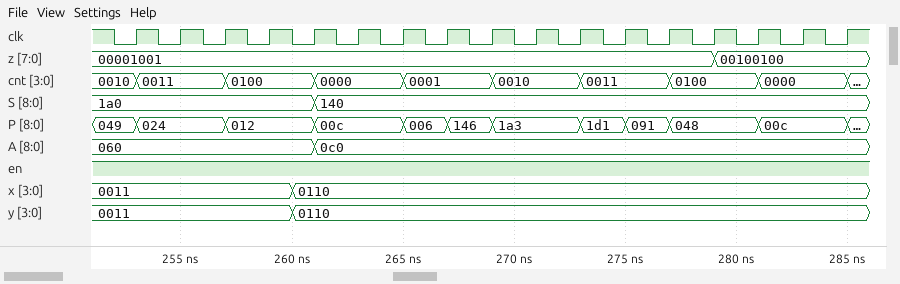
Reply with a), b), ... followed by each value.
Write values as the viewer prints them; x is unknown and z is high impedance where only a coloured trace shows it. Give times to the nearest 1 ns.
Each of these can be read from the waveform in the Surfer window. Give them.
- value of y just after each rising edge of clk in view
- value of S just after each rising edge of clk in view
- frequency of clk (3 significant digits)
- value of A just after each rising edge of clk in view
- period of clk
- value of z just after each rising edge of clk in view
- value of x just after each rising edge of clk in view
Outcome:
a) 0011, 0011, 0011, 0011, 0110, 0110, 0110, 0110, 0110, 0110, 0110, 0110, 0110, 0110, 0110, 0110, 0110
b) 1a0, 1a0, 1a0, 1a0, 140, 140, 140, 140, 140, 140, 140, 140, 140, 140, 140, 140, 140
c) 500 MHz
d) 060, 060, 060, 060, 0c0, 0c0, 0c0, 0c0, 0c0, 0c0, 0c0, 0c0, 0c0, 0c0, 0c0, 0c0, 0c0
e) 2 ns
f) 00001001, 00001001, 00001001, 00001001, 00001001, 00001001, 00001001, 00001001, 00001001, 00001001, 00001001, 00001001, 00001001, 00100100, 00100100, 00100100, 00100100
g) 0011, 0011, 0011, 0011, 0110, 0110, 0110, 0110, 0110, 0110, 0110, 0110, 0110, 0110, 0110, 0110, 0110
